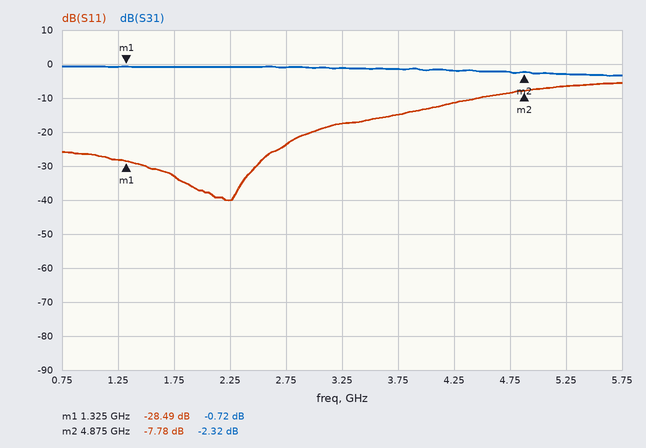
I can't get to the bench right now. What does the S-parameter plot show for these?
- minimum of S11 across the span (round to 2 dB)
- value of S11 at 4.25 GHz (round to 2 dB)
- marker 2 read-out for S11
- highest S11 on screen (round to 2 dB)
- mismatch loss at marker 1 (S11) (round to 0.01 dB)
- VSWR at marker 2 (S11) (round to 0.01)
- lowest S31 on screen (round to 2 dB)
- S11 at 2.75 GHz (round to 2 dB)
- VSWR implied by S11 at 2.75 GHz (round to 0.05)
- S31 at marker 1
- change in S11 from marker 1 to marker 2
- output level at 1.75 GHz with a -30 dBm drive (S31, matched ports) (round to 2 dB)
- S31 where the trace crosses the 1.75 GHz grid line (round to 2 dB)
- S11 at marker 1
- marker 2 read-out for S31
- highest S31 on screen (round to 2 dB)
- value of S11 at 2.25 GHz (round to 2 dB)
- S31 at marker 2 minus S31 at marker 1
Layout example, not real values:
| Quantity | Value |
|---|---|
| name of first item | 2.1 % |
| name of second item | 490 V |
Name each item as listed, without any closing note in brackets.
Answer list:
| Quantity | Value |
|---|---|
| minimum of S11 across the span | -40 dB |
| value of S11 at 4.25 GHz | -12 dB |
| marker 2 read-out for S11 | -7.78 dB |
| highest S11 on screen | -6 dB |
| mismatch loss at marker 1 (S11) | 0.01 dB |
| VSWR at marker 2 (S11) | 2.38 |
| lowest S31 on screen | -4 dB |
| S11 at 2.75 GHz | -24 dB |
| VSWR implied by S11 at 2.75 GHz | 1.15 |
| S31 at marker 1 | -0.72 dB |
| change in S11 from marker 1 to marker 2 | 20.71 dB |
| output level at 1.75 GHz with a -30 dBm drive (S31, matched ports) | -30 dBm |
| S31 where the trace crosses the 1.75 GHz grid line | 0 dB |
| S11 at marker 1 | -28.49 dB |
| marker 2 read-out for S31 | -2.32 dB |
| highest S31 on screen | 0 dB |
| value of S11 at 2.25 GHz | -40 dB |
| S31 at marker 2 minus S31 at marker 1 | -1.60 dB |
